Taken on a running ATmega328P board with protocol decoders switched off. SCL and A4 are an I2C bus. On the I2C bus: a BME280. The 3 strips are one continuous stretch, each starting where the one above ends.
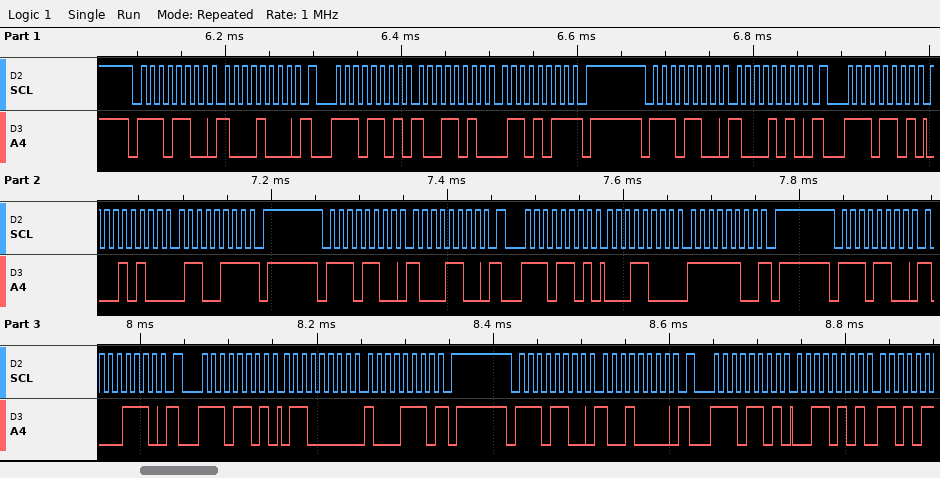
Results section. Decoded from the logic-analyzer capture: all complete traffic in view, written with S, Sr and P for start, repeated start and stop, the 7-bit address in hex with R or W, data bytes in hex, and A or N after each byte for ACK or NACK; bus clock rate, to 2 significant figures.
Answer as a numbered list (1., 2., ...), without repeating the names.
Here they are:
1. S 76W A 88 A Sr 76R A 9A A 6B N P S 76W A 8A A Sr 76R A 14 A 67 N P S 76W A 8C A Sr 76R A 18 A FC N P S 76W A 8E A Sr 76R A 60 A 8E N P S 76W A 90 A Sr 76R A 35 A
2. 100 kHz
